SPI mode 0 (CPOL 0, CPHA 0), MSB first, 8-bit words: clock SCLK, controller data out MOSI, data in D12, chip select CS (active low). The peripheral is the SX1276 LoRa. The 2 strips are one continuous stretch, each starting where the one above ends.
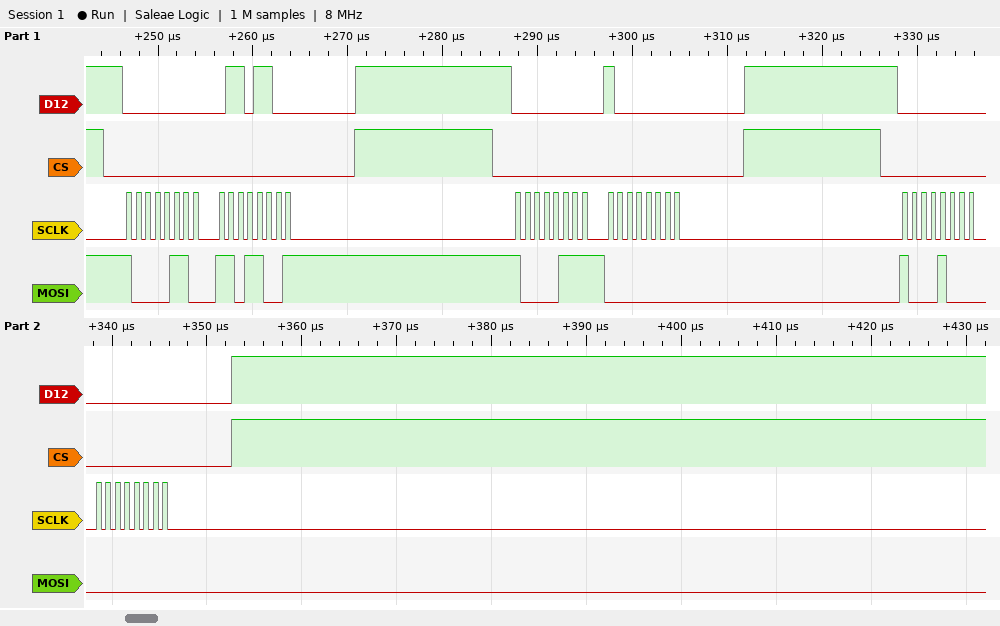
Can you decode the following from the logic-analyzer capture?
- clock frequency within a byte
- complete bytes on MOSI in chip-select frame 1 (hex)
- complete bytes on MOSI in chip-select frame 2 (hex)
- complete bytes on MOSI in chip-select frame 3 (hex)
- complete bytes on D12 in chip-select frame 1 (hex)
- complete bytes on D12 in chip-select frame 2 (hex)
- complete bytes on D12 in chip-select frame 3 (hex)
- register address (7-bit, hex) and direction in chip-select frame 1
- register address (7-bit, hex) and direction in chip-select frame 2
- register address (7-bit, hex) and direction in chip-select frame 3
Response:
1 MHz
86 D9
87 00
88 00
00 6C
00 80
00 00
0x06 write
0x07 write
0x08 write
